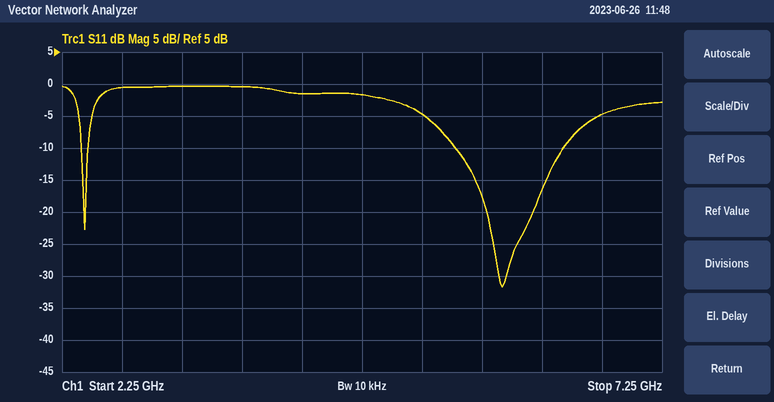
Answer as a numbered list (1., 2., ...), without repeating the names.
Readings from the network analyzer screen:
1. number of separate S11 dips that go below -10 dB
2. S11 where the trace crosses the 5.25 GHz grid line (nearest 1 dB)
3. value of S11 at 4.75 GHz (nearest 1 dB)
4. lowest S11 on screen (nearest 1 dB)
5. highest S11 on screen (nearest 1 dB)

1. 2
2. -5 dB
3. -2 dB
4. -32 dB
5. 0 dB
